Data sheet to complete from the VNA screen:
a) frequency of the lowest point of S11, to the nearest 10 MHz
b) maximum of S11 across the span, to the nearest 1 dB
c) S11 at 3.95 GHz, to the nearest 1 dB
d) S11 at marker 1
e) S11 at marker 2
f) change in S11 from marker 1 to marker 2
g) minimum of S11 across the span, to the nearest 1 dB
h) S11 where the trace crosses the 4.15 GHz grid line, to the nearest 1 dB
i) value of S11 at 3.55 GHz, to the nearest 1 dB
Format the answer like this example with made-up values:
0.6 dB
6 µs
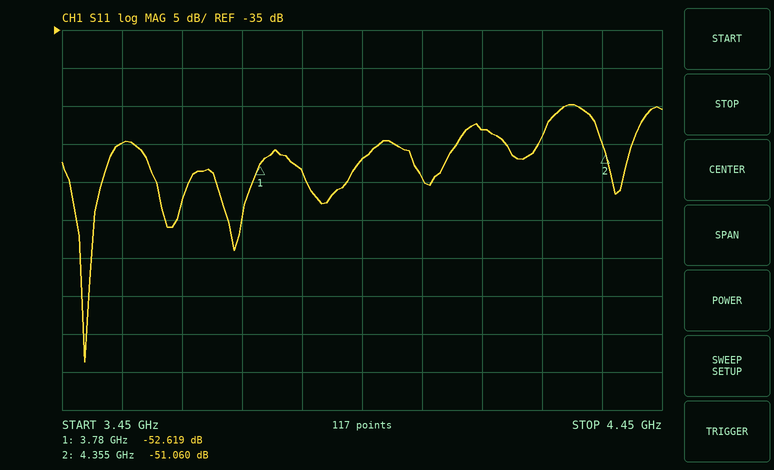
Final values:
3.49 GHz
-45 dB
-52 dB
-52.619 dB
-51.060 dB
1.559 dB
-79 dB
-48 dB
-50 dB
